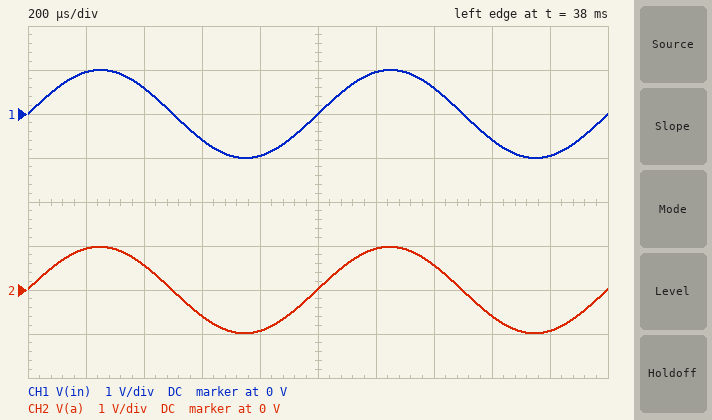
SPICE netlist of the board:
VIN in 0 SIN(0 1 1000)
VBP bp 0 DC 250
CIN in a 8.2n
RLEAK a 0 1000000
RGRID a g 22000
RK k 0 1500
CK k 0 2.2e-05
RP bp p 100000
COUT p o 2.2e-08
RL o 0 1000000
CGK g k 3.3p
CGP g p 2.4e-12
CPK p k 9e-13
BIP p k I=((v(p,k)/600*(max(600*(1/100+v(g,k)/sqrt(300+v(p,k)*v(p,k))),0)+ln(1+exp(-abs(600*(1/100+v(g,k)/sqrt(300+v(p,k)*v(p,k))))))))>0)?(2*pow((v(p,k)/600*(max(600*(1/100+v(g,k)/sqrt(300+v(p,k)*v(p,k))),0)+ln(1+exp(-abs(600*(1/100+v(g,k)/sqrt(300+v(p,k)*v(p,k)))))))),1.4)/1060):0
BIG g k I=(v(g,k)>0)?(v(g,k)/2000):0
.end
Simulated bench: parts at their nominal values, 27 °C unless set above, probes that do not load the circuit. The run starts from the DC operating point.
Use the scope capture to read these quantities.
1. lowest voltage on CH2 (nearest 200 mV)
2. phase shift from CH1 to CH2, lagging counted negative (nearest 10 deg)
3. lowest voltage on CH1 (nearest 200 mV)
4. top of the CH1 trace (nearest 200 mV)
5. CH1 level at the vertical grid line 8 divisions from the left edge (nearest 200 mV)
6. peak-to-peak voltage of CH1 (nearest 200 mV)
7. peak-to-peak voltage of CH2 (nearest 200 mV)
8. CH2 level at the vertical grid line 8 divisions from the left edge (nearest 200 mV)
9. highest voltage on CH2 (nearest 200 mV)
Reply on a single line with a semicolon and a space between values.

-1.0 V; 0 deg; -1.0 V; 1.0 V; -600 mV; 2.0 V; 2.0 V; -600 mV; 1.0 V
